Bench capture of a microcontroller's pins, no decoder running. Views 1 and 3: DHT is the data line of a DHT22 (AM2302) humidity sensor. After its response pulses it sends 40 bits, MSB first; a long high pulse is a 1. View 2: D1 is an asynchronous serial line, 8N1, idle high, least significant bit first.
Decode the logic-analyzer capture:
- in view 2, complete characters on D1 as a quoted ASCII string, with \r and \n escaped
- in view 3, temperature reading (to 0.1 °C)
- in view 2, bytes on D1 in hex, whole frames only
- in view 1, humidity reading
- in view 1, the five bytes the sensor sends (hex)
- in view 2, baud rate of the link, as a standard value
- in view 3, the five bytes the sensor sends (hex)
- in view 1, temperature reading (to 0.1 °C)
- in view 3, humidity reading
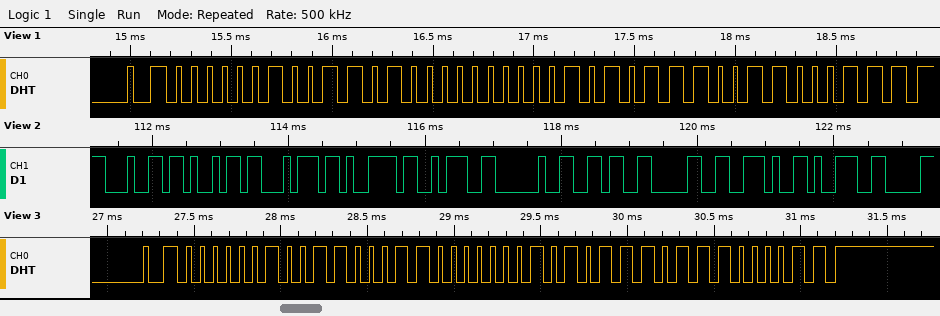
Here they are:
"dity: 60.9"
34.9 °C
64 69 74 79 3A 20 36 30 2E 39
61.6 %
02 68 01 5C C7
9600 baud
02 63 01 5D C3
34.8 °C
61.1 %
